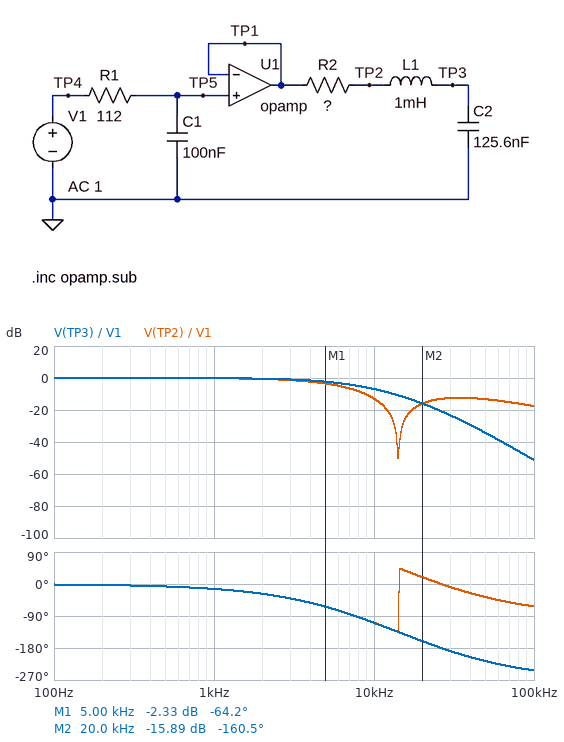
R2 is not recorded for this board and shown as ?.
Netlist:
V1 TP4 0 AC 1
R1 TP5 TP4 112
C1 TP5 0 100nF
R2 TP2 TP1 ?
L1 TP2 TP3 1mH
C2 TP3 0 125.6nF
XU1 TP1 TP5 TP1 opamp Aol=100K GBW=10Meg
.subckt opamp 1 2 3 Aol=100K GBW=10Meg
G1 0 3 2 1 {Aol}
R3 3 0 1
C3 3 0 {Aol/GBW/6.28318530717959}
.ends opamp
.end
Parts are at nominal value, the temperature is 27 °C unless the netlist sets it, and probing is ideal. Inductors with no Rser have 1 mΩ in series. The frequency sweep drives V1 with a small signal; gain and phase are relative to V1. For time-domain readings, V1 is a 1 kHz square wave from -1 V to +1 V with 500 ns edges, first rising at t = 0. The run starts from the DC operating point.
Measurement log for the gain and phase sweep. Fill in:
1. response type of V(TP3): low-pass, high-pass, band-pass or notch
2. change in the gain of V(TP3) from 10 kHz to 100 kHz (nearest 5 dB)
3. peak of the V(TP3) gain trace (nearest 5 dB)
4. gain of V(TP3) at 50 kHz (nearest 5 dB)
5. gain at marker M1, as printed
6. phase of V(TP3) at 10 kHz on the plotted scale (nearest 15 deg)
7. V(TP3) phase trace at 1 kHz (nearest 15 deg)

low-pass
-45 dB
0 dB
-35 dB
-2.33 dB
-105 deg
-15 deg
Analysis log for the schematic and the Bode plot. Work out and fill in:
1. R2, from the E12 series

220 Ω
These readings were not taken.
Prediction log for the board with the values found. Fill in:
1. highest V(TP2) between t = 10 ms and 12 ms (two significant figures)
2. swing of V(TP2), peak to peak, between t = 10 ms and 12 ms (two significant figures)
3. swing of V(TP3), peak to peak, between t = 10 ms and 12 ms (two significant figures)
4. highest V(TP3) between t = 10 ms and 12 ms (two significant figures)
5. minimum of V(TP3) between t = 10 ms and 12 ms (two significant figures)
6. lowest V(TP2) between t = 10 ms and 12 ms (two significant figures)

1.0 V
2.0 V
2.0 V
1.0 V
-1.0 V
-1.0 V
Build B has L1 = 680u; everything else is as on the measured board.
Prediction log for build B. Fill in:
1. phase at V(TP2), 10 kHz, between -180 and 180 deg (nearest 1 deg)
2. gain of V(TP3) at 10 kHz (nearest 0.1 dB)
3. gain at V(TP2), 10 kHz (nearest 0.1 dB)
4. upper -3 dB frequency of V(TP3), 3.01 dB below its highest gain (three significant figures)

-104 deg
-7.1 dB
-10.7 dB
5.56 kHz
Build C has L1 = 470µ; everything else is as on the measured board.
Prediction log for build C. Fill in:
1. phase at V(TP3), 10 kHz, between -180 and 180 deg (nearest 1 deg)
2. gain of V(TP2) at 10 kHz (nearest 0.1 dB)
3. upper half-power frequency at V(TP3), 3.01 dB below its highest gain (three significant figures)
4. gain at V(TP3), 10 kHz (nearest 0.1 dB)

-101 deg
-9.6 dB
5.40 kHz
-7.3 dB
